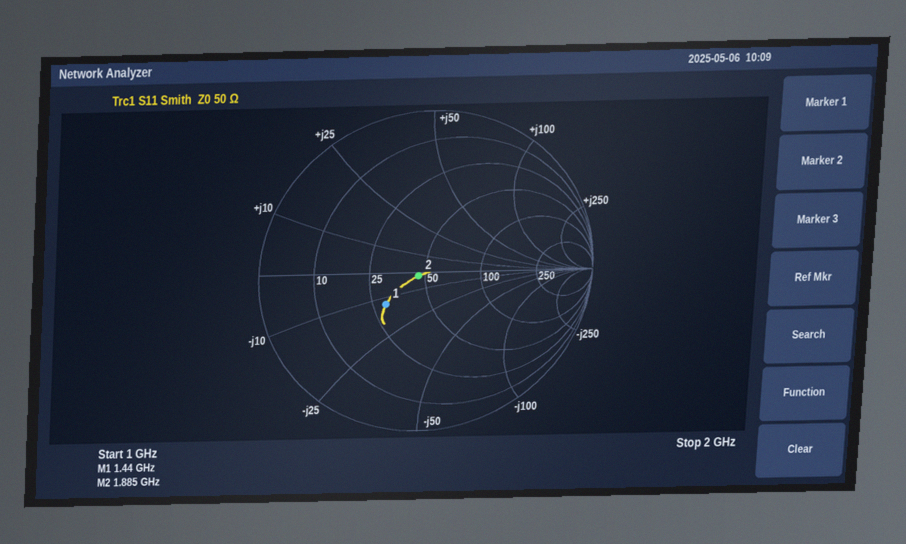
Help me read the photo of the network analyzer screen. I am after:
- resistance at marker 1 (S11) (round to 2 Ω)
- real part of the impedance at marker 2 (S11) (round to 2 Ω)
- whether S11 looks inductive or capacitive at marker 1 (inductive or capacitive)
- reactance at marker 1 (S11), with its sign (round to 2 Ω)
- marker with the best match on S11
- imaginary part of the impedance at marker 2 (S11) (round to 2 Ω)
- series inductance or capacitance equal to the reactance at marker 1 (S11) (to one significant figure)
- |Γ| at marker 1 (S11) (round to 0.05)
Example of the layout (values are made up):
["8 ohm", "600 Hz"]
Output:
["30 Ω", "46 Ω", "capacitive", "-12 Ω", "marker 2", "-2 Ω", "9 pF", "0.30"]
